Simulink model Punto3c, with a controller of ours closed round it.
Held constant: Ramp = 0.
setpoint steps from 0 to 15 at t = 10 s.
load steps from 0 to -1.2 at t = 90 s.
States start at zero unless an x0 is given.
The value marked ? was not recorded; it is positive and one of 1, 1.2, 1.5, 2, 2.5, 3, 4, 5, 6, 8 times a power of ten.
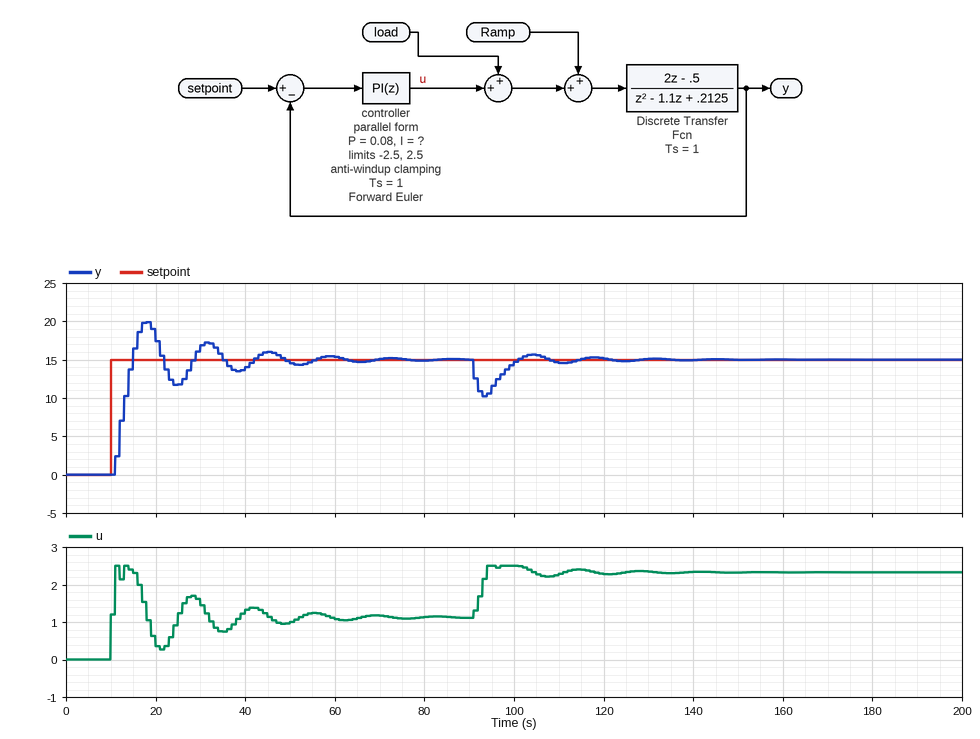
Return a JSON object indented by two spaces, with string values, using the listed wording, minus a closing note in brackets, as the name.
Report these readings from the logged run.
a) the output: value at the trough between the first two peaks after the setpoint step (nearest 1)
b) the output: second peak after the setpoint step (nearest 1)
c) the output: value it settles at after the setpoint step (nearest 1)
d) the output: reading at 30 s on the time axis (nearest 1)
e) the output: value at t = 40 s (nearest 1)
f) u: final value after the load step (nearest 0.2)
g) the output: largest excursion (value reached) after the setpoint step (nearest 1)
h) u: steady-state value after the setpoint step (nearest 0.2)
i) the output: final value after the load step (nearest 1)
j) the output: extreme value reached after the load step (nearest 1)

{
  "the output: value at the trough between the first two peaks after the setpoint step": "12",
  "the output: second peak after the setpoint step": "17",
  "the output: value it settles at after the setpoint step": "15",
  "the output: reading at 30 s on the time axis": "17",
  "the output: value at t = 40 s": "14",
  "u: final value after the load step": "2.4",
  "the output: largest excursion (value reached) after the setpoint step": "20",
  "u: steady-state value after the setpoint step": "1.2",
  "the output: final value after the load step": "15",
  "the output: extreme value reached after the load step": "10"
}
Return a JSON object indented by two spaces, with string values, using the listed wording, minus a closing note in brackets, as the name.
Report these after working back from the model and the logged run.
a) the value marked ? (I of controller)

{
  "the value marked ?": "0.1"
}
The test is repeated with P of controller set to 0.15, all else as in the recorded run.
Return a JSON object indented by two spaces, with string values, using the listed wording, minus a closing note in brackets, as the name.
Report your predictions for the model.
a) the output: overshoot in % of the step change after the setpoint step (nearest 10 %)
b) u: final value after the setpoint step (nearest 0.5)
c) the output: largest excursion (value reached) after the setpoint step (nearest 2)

{
  "the output: overshoot in % of the step change after the setpoint step": "20 %",
  "u: final value after the setpoint step": "1.0",
  "the output: largest excursion (value reached) after the setpoint step": "18"
}
